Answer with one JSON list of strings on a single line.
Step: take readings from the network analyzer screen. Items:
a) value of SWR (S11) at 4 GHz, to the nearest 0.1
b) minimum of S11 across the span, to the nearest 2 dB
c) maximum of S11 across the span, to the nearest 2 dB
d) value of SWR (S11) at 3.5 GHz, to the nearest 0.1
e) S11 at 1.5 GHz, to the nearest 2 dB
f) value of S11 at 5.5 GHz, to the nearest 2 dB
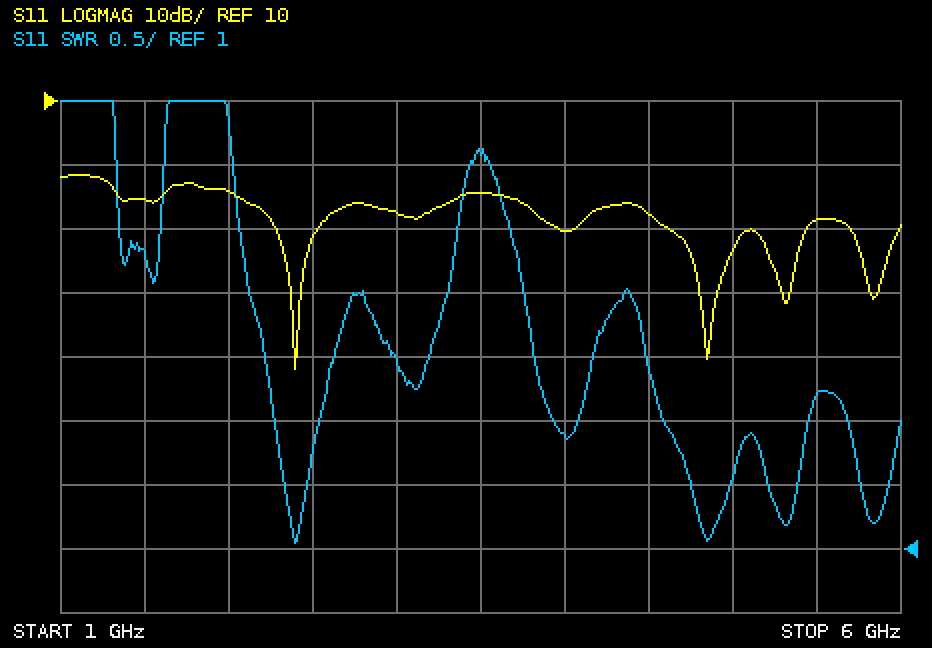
["1.9", "-32 dB", "-2 dB", "4.1", "-6 dB", "-8 dB"]
